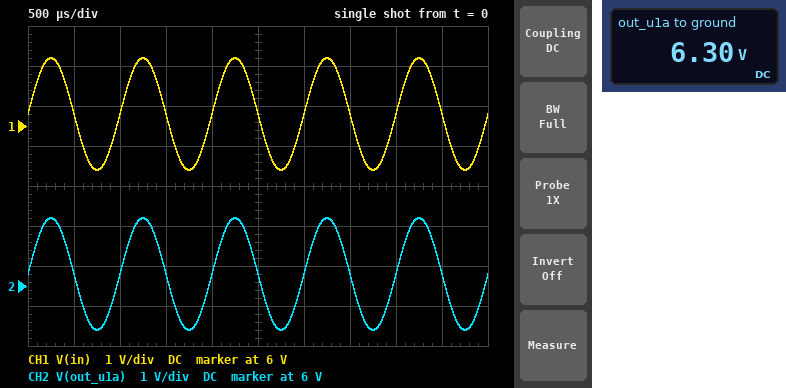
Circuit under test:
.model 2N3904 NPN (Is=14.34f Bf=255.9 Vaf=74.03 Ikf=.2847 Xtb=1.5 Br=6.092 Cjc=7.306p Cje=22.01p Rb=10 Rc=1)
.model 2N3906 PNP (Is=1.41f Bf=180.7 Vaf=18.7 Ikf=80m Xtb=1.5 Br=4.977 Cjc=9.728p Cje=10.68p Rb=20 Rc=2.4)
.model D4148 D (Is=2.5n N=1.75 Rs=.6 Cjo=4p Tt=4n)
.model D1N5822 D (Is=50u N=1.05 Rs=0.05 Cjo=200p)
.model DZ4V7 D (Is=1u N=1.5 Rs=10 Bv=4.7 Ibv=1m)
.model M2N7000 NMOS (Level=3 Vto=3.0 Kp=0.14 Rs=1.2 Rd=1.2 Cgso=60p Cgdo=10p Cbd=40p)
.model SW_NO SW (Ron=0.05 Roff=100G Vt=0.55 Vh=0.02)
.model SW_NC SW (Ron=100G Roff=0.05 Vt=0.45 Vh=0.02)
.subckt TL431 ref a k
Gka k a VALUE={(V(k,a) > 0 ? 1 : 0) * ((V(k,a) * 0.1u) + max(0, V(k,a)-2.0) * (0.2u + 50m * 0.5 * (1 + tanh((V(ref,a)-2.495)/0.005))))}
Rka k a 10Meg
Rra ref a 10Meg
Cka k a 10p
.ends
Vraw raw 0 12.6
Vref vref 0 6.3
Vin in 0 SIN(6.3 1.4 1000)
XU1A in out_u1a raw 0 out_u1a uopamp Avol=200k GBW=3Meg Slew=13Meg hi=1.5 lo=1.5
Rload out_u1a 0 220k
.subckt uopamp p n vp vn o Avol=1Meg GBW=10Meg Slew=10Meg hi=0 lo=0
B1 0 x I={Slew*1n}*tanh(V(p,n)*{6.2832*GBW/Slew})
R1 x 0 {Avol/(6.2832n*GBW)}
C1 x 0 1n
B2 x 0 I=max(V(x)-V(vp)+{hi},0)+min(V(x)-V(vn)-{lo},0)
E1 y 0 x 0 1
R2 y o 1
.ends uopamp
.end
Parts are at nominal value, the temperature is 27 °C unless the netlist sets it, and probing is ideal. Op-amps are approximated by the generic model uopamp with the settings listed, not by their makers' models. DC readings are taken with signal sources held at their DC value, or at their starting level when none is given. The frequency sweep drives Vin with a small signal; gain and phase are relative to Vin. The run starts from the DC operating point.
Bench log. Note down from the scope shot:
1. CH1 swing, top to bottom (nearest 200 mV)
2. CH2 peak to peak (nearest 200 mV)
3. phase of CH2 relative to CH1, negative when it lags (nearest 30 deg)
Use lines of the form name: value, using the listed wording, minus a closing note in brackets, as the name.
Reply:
CH1 swing, top to bottom: 2.8 V
CH2 peak to peak: 2.8 V
phase of CH2 relative to CH1, negative when it lags: 0 deg
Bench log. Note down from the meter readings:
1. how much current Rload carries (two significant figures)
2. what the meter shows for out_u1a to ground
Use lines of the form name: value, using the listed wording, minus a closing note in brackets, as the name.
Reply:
how much current Rload carries: 29 µA
what the meter shows for out_u1a to ground: 6.30 V
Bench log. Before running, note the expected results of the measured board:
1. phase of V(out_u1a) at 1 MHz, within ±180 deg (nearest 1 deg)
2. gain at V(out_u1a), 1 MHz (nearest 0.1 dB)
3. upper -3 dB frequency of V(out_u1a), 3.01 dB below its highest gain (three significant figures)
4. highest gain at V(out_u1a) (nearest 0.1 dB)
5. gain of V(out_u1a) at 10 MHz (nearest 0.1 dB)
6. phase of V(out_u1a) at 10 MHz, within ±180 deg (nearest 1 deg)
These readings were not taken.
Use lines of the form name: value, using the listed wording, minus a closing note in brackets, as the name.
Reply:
phase of V(out_u1a) at 1 MHz, within ±180 deg: -18 deg
gain at V(out_u1a), 1 MHz: -0.5 dB
upper -3 dB frequency of V(out_u1a), 3.01 dB below its highest gain: 3.00 MHz
highest gain at V(out_u1a): 0 dB
gain of V(out_u1a) at 10 MHz: -10.8 dB
phase of V(out_u1a) at 10 MHz, within ±180 deg: -73 deg
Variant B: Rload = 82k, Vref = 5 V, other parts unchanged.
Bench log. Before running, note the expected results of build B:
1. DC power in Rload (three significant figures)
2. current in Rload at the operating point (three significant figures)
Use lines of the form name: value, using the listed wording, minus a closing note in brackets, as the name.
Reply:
DC power in Rload: 484 µW
current in Rload at the operating point: 76.8 µA
